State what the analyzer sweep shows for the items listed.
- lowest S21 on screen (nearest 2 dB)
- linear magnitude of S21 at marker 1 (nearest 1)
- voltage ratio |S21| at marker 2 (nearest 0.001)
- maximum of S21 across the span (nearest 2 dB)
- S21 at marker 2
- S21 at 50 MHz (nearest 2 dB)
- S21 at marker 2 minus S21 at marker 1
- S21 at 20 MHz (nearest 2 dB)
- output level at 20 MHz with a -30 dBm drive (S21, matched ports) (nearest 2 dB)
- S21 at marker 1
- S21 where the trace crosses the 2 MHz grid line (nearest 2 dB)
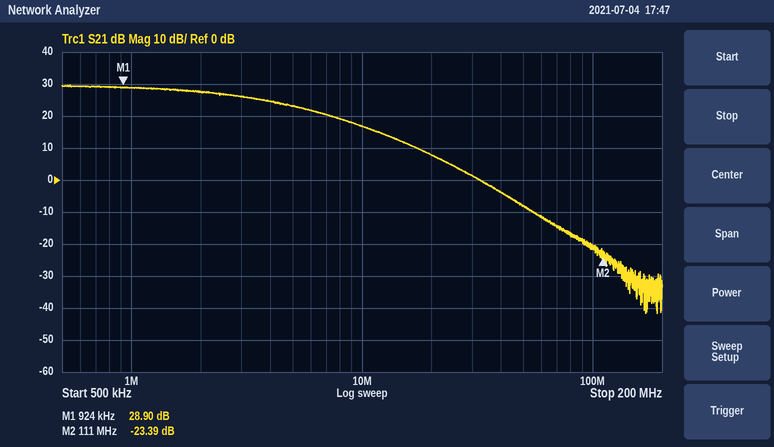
-42 dB
28
0.068
30 dB
-23.39 dB
-8 dB
-52.29 dB
8 dB
-22 dBm
28.90 dB
28 dB
